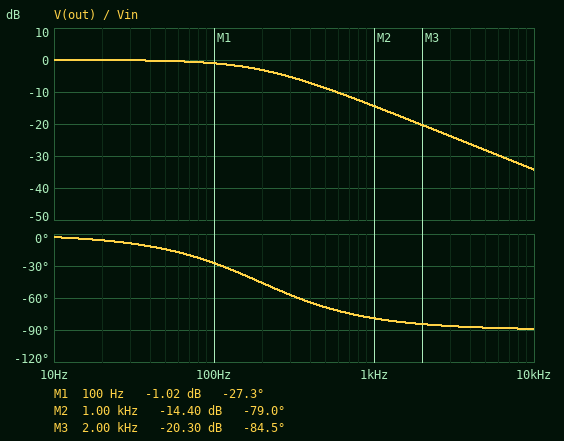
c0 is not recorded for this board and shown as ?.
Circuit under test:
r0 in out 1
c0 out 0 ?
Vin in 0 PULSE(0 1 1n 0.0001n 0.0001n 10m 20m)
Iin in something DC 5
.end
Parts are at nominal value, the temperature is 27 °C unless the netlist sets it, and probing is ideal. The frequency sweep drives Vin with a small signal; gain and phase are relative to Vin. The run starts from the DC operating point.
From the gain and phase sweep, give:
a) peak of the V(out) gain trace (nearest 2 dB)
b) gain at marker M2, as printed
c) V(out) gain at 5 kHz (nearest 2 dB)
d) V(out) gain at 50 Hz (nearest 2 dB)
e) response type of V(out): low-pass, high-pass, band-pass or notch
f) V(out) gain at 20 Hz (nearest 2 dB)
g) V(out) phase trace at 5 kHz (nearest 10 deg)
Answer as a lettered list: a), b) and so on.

a) 0 dB
b) -14.40 dB
c) -28 dB
d) 0 dB
e) low-pass
f) 0 dB
g) -90 deg
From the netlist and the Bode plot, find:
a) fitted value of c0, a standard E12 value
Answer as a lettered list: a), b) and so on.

a) 820 µF
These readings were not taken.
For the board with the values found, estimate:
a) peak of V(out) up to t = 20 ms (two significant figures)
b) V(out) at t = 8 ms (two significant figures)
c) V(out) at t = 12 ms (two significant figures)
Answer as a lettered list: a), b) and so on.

a) 1.0 V
b) 1.0 V
c) 87 mV
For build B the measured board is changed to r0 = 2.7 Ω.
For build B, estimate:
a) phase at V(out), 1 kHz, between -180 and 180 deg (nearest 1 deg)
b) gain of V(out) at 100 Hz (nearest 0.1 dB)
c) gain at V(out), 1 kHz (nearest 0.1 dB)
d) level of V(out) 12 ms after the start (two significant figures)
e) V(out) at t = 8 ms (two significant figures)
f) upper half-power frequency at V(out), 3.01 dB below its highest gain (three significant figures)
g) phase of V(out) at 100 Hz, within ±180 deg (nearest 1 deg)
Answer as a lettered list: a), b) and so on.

a) -86 deg
b) -4.7 dB
c) -22.9 dB
d) 400 mV
e) 970 mV
f) 71.9 Hz
g) -54 deg
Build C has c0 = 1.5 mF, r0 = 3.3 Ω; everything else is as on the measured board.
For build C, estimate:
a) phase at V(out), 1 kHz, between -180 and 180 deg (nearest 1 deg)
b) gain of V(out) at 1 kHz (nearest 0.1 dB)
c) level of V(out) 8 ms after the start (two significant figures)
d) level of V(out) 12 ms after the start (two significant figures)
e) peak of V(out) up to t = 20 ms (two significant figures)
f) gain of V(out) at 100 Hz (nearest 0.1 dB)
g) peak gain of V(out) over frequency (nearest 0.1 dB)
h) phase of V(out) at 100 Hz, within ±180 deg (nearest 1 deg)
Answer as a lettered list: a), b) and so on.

a) -88 deg
b) -29.9 dB
c) 800 mV
d) 580 mV
e) 870 mV
f) -10.3 dB
g) 0 dB
h) -72 deg
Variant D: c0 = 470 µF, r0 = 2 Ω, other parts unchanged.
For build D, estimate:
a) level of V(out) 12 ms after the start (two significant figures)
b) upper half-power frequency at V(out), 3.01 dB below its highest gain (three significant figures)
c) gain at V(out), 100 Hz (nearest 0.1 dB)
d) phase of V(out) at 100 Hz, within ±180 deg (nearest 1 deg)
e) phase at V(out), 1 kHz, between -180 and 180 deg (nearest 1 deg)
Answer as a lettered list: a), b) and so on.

a) 120 mV
b) 169 Hz
c) -1.3 dB
d) -31 deg
e) -80 deg
